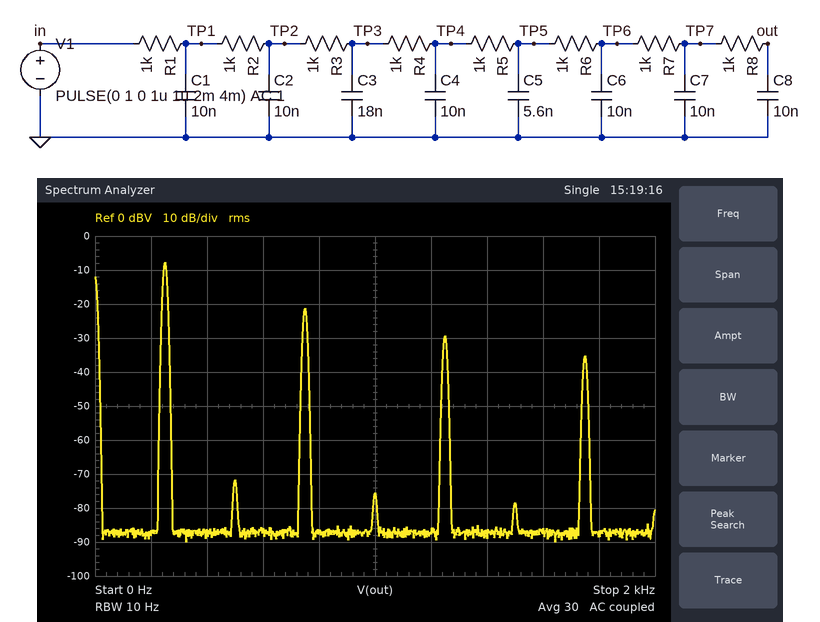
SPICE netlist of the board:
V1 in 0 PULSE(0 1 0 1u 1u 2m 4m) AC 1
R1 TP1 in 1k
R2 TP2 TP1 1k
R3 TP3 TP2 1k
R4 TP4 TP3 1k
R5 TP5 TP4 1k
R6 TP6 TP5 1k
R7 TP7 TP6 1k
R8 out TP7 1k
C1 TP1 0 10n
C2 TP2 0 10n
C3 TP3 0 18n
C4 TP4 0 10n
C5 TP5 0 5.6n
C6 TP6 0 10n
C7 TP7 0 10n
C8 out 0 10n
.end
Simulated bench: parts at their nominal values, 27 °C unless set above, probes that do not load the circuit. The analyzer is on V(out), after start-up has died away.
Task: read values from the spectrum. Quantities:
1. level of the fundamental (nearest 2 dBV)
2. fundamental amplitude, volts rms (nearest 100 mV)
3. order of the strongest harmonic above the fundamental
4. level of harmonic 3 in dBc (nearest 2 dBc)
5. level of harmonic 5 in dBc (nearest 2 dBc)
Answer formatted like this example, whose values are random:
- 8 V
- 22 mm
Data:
- -8 dBV
- 400 mV
- 3
- -14 dBc
- -22 dBc
